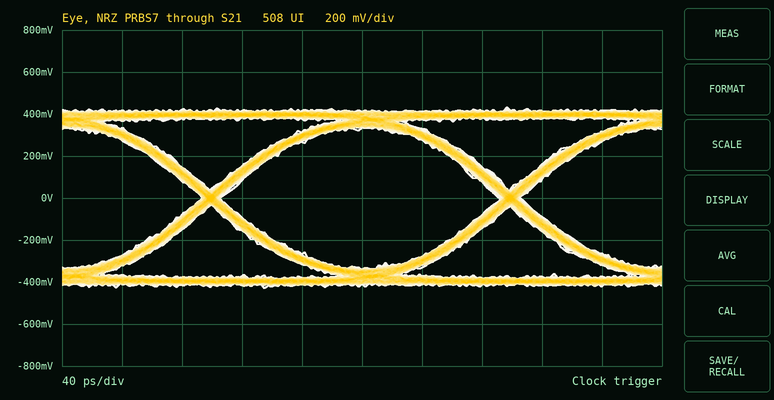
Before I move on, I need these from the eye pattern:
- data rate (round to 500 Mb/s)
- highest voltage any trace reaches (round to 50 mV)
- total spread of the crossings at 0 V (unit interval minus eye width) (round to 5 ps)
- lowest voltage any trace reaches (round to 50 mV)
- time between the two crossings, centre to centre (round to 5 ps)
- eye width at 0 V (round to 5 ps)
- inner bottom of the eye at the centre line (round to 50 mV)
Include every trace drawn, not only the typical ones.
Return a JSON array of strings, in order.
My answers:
["5.0 Gb/s", "450 mV", "15 ps", "-450 mV", "200 ps", "185 ps", "-350 mV"]
